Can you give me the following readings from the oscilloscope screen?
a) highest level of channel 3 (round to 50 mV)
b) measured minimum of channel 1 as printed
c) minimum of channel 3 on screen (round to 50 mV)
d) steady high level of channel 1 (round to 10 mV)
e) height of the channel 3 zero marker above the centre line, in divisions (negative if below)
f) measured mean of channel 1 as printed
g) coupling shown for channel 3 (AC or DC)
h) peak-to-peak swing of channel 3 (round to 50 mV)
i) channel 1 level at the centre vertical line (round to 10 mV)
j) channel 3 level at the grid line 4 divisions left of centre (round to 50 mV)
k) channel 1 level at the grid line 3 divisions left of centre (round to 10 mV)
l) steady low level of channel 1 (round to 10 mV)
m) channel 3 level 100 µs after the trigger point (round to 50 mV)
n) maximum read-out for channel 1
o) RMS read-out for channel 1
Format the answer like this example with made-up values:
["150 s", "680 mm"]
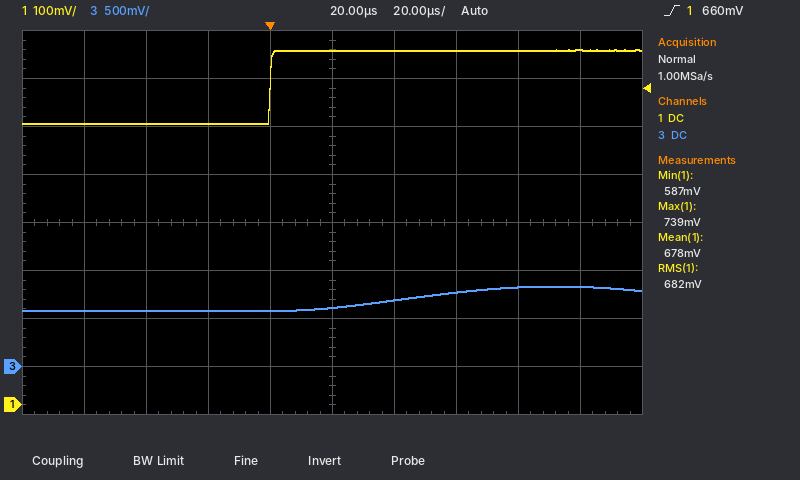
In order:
["850 mV", "587 mV", "600 mV", "740 mV", "-3.0 div", "678 mV", "DC", "250 mV", "740 mV", "600 mV", "590 mV", "590 mV", "850 mV", "739 mV", "682 mV"]
